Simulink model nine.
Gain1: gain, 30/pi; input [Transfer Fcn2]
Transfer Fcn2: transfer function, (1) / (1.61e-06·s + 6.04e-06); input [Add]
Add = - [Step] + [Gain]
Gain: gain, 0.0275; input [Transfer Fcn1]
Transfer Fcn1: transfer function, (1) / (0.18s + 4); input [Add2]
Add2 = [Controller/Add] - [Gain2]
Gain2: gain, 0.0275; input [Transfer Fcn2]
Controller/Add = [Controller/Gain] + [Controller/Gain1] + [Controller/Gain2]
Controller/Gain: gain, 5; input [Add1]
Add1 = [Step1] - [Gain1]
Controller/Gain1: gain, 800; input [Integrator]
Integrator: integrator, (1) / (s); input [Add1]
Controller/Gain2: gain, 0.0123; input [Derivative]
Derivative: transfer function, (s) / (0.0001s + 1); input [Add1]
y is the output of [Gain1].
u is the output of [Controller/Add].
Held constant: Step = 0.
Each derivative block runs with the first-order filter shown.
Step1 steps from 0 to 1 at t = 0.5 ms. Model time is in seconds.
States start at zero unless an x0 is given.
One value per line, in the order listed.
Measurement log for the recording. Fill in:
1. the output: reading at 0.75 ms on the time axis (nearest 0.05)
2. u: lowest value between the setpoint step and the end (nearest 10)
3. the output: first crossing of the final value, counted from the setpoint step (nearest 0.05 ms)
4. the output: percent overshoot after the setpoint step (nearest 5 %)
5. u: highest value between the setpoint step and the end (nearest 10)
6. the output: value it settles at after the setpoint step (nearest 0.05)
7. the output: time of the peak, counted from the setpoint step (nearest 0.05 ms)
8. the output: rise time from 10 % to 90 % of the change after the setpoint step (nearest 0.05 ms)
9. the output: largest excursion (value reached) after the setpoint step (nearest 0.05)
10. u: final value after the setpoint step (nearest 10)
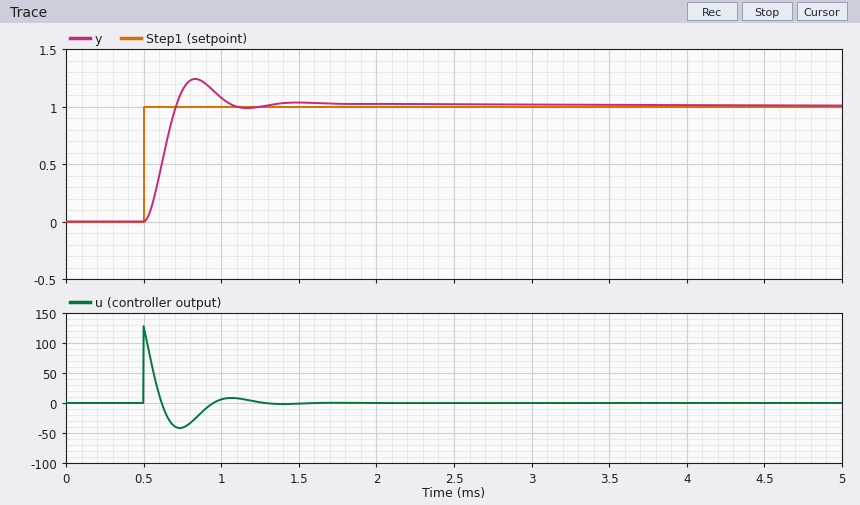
1.15
-40
0.20 ms
25 %
130
1.00
0.35 ms
0.15 ms
1.25
0
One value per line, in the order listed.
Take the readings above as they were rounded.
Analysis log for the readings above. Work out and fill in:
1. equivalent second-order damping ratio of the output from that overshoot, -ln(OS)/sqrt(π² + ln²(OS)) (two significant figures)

0.40
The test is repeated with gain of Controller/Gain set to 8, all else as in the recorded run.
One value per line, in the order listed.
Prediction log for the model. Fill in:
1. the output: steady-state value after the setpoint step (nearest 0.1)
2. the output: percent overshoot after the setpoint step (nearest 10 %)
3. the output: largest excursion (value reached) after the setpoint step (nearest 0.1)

1.0
30 %
1.3
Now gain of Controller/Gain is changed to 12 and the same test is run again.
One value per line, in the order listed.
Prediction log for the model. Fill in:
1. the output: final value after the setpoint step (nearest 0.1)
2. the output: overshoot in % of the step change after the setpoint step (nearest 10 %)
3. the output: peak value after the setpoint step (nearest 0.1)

1.0
30 %
1.3
